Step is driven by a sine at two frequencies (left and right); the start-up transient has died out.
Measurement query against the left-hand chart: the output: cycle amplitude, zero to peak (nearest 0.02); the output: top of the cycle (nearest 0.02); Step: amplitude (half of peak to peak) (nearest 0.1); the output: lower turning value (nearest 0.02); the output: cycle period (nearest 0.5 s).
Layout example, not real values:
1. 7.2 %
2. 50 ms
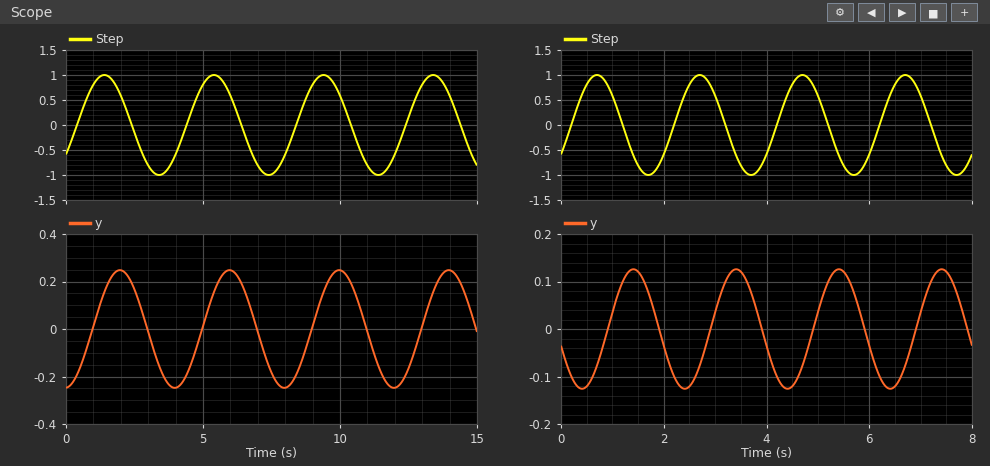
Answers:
1. 0.24
2. 0.24
3. 1.0
4. -0.24
5. 4.0 s
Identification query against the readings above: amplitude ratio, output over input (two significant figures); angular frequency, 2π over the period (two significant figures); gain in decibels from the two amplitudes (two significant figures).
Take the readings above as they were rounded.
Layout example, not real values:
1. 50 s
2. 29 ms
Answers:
1. 0.24
2. 1.6 rad/s
3. -12 dB
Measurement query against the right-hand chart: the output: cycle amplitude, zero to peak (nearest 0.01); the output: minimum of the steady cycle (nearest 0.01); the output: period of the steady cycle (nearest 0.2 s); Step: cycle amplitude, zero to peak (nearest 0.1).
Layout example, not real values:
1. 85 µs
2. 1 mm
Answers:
1. 0.13
2. -0.13
3. 2.0 s
4. 1.0
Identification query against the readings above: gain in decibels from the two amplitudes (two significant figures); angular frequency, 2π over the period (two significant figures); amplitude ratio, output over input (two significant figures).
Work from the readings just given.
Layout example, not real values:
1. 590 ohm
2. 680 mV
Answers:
1. -18 dB
2. 3.1 rad/s
3. 0.13
